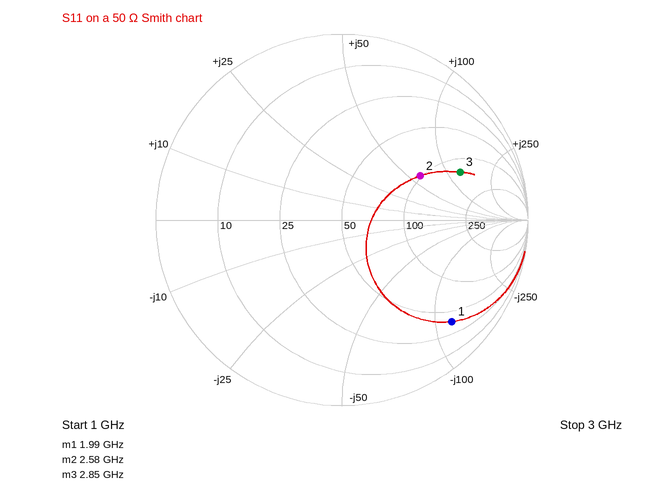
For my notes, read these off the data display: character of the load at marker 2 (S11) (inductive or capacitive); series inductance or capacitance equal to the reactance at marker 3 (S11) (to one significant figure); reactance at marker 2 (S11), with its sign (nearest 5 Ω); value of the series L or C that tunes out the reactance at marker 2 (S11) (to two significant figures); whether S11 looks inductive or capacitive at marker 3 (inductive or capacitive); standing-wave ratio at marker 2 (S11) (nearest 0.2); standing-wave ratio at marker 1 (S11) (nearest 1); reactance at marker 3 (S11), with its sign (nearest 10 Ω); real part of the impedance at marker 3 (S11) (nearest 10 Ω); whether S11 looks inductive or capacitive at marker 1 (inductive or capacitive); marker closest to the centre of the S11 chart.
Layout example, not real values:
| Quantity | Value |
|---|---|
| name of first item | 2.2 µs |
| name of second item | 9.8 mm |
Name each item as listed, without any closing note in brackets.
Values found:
| Quantity | Value |
|---|---|
| character of the load at marker 2 (S11) | inductive |
| series inductance or capacitance equal to the reactance at marker 3 (S11) | 7 nH |
| reactance at marker 2 (S11), with its sign | +60 Ω |
| value of the series L or C that tunes out the reactance at marker 2 (S11) | 1.0 pF |
| whether S11 looks inductive or capacitive at marker 3 | inductive |
| standing-wave ratio at marker 2 (S11) | 2.8 |
| standing-wave ratio at marker 1 (S11) | 9 |
| reactance at marker 3 (S11), with its sign | +130 Ω |
| real part of the impedance at marker 3 (S11) | 130 Ω |
| whether S11 looks inductive or capacitive at marker 1 | capacitive |
| marker closest to the centre of the S11 chart | marker 2 |
